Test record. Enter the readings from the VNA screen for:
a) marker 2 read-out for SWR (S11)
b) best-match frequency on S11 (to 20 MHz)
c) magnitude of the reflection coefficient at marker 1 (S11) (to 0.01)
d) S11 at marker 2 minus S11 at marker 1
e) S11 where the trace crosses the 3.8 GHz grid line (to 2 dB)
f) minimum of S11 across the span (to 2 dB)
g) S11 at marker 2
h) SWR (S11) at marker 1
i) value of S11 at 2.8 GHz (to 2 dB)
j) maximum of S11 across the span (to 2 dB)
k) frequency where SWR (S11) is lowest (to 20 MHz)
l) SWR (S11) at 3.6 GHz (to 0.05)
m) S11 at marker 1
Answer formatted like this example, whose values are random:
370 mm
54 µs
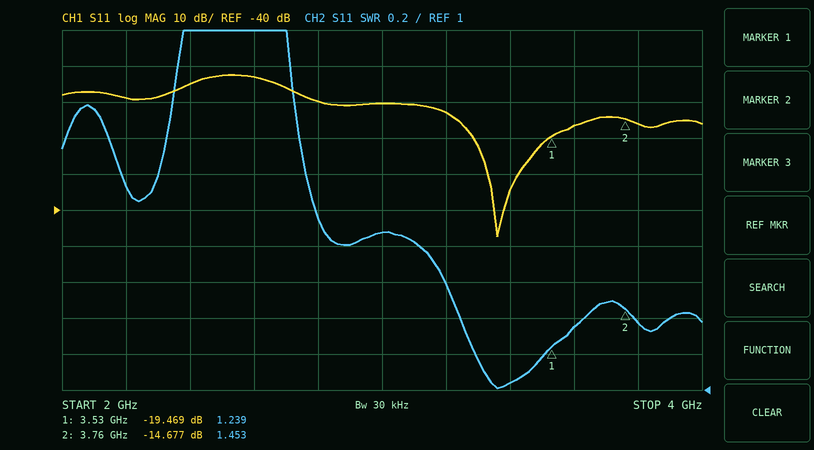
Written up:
1.453
3.36 GHz
0.11
4.792 dB
-16 dB
-48 dB
-14.677 dB
1.239
-10 dB
-2 dB
3.36 GHz
1.35
-19.469 dB
